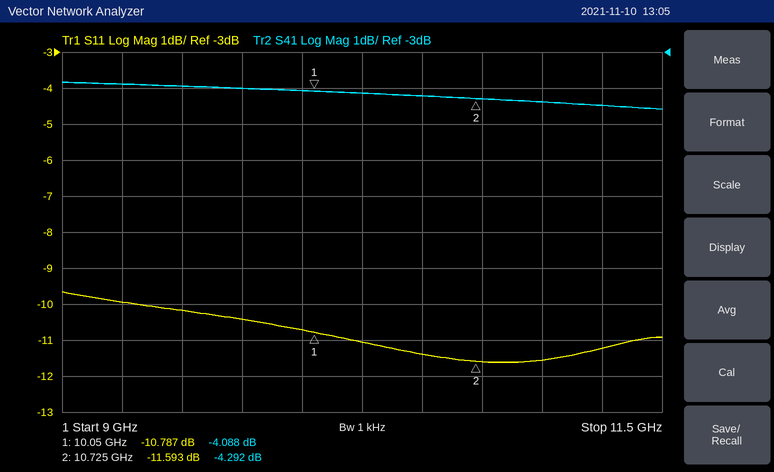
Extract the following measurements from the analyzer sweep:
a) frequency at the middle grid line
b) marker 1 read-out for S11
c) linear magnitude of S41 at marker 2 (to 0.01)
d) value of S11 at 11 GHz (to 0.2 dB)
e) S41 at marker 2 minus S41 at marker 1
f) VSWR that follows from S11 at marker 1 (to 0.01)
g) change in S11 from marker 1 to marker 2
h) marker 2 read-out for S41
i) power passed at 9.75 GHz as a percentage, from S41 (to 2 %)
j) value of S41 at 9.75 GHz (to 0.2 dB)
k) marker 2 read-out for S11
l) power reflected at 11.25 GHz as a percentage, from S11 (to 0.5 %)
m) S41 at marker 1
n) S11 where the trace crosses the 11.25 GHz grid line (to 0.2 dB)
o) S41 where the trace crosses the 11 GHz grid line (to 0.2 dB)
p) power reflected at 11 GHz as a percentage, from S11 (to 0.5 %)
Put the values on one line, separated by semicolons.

10.25 GHz; -10.787 dB; 0.61; -11.6 dB; -0.204 dB; 1.81; -0.806 dB; -4.292 dB; 40 %; -4.0 dB; -11.593 dB; 7.5 %; -4.088 dB; -11.2 dB; -4.4 dB; 7.0 %
